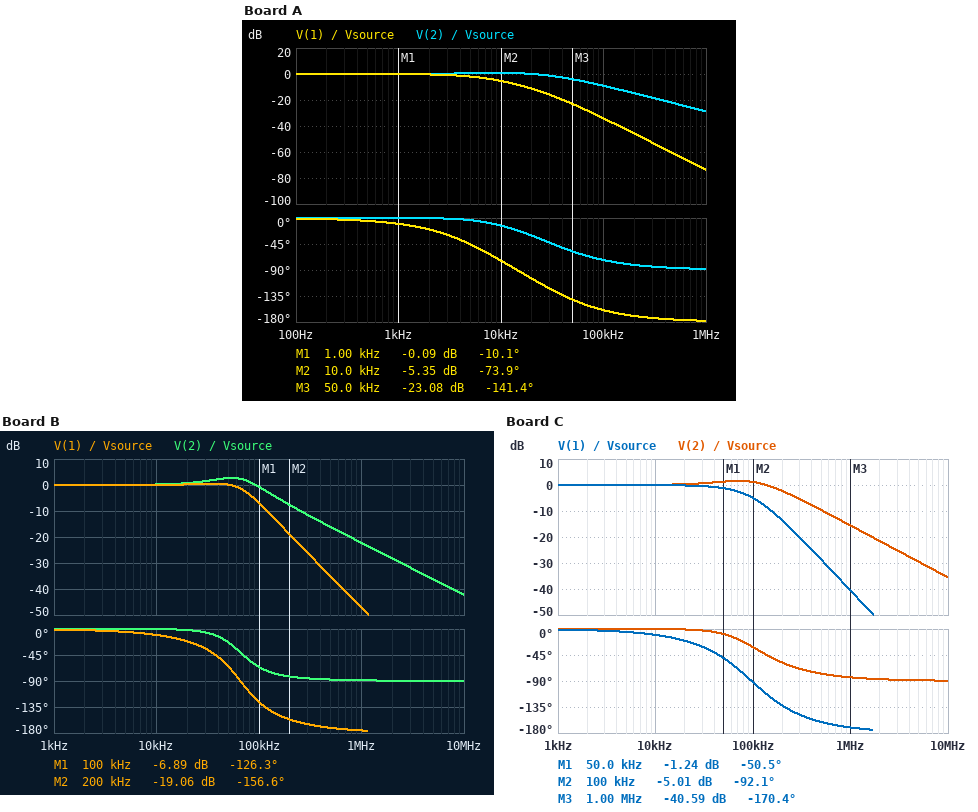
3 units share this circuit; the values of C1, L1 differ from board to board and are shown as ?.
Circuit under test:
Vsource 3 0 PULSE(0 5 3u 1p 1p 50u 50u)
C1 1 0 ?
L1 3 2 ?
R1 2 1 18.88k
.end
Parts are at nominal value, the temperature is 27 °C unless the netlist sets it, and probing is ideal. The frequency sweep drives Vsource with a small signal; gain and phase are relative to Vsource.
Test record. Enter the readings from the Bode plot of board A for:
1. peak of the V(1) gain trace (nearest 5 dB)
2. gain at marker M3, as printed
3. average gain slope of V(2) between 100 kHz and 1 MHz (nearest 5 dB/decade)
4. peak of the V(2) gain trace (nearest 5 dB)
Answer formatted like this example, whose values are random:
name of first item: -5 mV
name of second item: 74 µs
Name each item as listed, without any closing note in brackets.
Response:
peak of the V(1) gain trace: 0 dB
gain at marker M3, as printed: -23.08 dB
average gain slope of V(2) between 100 kHz and 1 MHz: -20 dB/decade
peak of the V(2) gain trace: 0 dB
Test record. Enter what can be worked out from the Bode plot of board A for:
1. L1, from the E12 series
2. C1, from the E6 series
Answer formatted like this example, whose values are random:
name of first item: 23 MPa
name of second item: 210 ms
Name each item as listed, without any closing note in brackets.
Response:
L1, from the E12 series: 82 mH
C1, from the E6 series: 1.5 nF
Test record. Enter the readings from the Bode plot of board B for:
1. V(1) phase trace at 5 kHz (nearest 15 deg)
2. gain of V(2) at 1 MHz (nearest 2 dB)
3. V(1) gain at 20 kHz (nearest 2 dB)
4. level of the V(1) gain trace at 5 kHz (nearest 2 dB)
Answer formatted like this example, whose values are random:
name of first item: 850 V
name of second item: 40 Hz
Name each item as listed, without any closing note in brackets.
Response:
V(1) phase trace at 5 kHz: 0 deg
gain of V(2) at 1 MHz: -22 dB
V(1) gain at 20 kHz: 0 dB
level of the V(1) gain trace at 5 kHz: 0 dB
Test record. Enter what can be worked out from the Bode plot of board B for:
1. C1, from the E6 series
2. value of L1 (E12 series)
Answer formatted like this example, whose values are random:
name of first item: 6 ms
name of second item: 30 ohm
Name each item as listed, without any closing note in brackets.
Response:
C1, from the E6 series: 150 pF
value of L1: 39 mH
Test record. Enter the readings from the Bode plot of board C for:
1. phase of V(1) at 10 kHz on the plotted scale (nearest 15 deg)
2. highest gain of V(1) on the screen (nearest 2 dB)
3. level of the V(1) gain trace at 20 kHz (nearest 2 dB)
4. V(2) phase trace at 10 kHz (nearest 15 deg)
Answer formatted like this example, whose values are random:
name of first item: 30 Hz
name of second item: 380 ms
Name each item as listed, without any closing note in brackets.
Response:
phase of V(1) at 10 kHz on the plotted scale: -15 deg
highest gain of V(1) on the screen: 0 dB
level of the V(1) gain trace at 20 kHz: 0 dB
V(2) phase trace at 10 kHz: 0 deg
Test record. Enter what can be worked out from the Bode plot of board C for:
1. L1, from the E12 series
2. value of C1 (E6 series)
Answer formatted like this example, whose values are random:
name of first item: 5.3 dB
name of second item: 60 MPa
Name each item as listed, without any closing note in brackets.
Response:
L1, from the E12 series: 18 mH
value of C1: 150 pF
